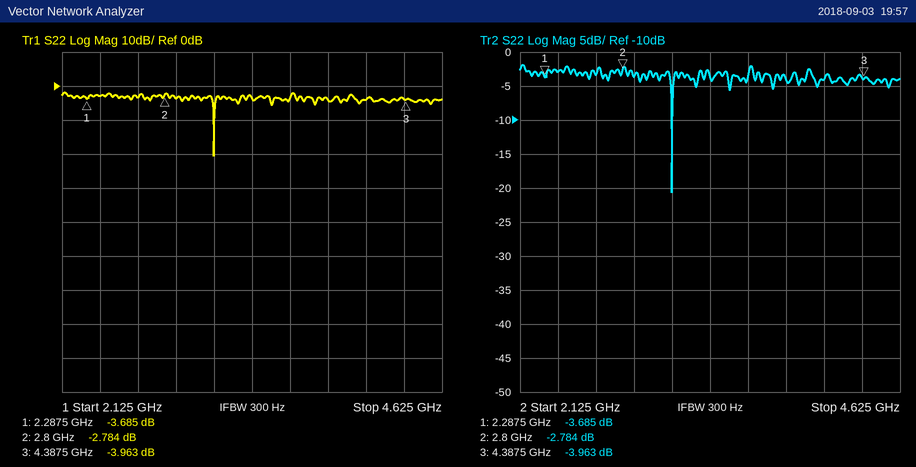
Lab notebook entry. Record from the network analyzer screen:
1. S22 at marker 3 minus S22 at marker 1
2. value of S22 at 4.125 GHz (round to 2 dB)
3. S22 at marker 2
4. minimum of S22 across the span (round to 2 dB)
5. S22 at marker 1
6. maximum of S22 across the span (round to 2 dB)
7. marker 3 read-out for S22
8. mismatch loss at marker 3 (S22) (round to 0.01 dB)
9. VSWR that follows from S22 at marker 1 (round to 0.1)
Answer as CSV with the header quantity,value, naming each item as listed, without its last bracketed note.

quantity,value
S22 at marker 3 minus S22 at marker 1,-0.278 dB
value of S22 at 4.125 GHz,-4 dB
S22 at marker 2,-2.784 dB
minimum of S22 across the span,-20 dB
S22 at marker 1,-3.685 dB
maximum of S22 across the span,-2 dB
marker 3 read-out for S22,-3.963 dB
mismatch loss at marker 3 (S22),2.23 dB
VSWR that follows from S22 at marker 1,4.8
